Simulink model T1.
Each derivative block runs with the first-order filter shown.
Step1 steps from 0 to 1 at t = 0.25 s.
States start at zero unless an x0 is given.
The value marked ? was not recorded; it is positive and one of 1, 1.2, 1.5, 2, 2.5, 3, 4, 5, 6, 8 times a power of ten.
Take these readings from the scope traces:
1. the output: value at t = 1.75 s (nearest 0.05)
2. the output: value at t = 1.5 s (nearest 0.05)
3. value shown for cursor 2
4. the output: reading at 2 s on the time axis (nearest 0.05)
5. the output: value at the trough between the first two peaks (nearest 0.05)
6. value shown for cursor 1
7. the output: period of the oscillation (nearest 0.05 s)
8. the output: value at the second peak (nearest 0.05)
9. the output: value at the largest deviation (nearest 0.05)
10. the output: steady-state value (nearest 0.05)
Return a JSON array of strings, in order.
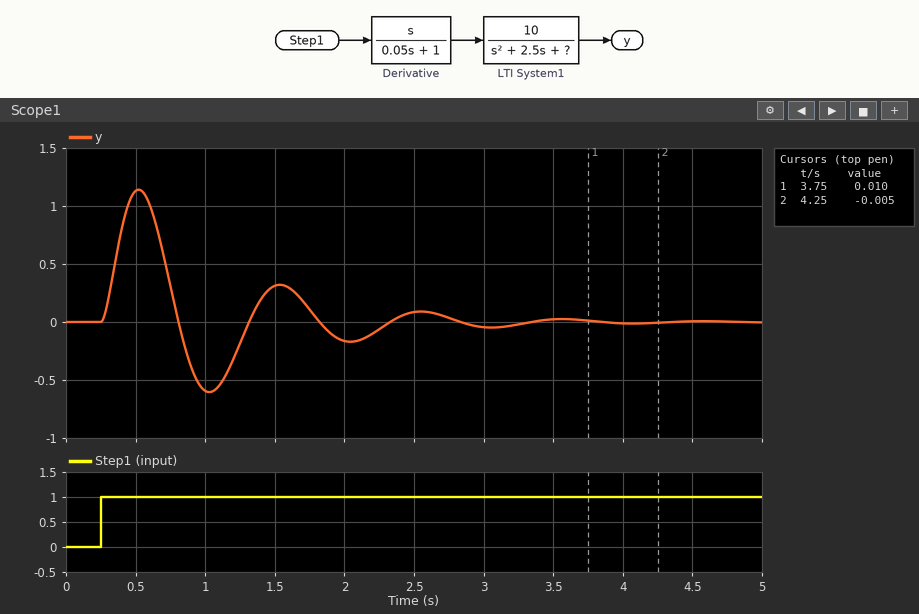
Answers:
["0.10", "0.30", "-0.005", "-0.15", "-0.60", "0.010", "1.00 s", "0.30", "1.15", "0.00"]
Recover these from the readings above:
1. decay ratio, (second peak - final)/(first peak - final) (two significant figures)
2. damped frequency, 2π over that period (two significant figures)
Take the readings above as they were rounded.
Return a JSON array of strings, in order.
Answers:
["0.26", "6.3 rad/s"]
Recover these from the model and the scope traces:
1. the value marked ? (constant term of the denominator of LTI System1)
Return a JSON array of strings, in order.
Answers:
["40"]
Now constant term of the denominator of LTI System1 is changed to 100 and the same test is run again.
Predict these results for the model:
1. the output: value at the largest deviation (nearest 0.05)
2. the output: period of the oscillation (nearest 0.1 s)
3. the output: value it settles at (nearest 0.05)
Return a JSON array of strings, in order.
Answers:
["0.75", "0.6 s", "0.00"]
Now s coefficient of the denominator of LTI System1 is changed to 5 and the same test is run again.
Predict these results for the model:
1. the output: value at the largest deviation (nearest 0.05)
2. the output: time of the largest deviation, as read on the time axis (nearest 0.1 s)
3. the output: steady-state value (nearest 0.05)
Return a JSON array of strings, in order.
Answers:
["0.90", "0.5 s", "0.00"]
